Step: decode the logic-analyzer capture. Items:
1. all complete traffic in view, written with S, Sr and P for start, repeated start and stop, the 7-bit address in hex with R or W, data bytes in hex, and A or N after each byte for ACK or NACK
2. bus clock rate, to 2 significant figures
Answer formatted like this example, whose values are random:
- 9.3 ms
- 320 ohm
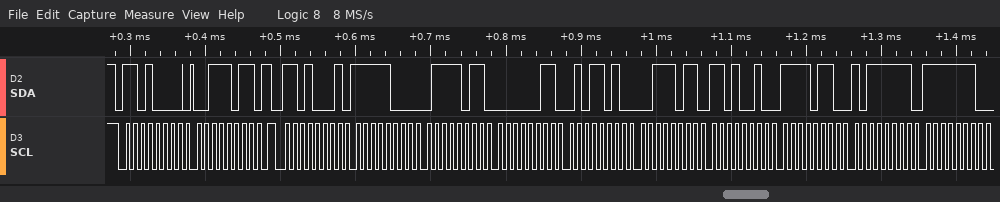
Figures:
- S 68W A 3B A Sr 68R A F8 A 7B A 03 A 5A A 3B A D2 A F6 A BF A FE A
- 100 kHz
